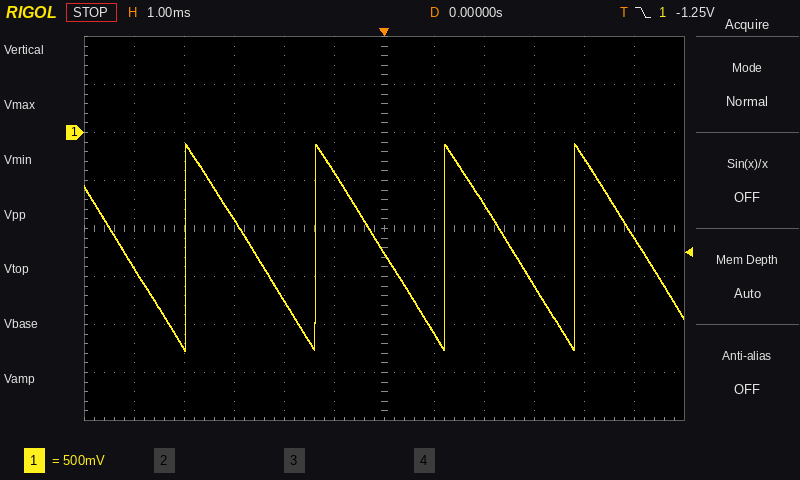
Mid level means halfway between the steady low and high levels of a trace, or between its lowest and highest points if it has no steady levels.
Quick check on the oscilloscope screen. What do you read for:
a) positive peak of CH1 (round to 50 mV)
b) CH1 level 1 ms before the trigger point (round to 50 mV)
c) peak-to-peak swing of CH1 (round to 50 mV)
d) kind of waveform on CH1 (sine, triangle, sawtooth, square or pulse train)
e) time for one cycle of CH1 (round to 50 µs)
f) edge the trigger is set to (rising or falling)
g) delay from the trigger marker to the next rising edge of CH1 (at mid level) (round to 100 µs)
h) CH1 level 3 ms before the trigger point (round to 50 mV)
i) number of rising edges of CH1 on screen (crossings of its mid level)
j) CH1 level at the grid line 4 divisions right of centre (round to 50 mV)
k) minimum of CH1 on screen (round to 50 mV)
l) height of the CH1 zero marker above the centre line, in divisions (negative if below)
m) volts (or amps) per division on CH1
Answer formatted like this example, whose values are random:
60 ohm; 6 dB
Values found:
-100 mV; -400 mV; 2.15 V; sawtooth; 2.60 ms; falling; 1.2 ms; -900 mV; 4; -250 mV; -2.25 V; +2.0 div; 500 mV
